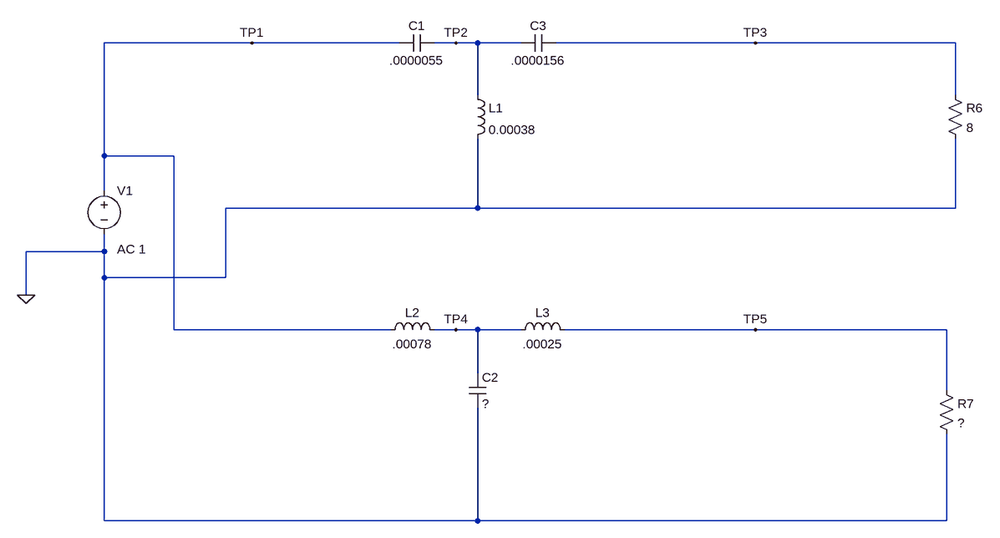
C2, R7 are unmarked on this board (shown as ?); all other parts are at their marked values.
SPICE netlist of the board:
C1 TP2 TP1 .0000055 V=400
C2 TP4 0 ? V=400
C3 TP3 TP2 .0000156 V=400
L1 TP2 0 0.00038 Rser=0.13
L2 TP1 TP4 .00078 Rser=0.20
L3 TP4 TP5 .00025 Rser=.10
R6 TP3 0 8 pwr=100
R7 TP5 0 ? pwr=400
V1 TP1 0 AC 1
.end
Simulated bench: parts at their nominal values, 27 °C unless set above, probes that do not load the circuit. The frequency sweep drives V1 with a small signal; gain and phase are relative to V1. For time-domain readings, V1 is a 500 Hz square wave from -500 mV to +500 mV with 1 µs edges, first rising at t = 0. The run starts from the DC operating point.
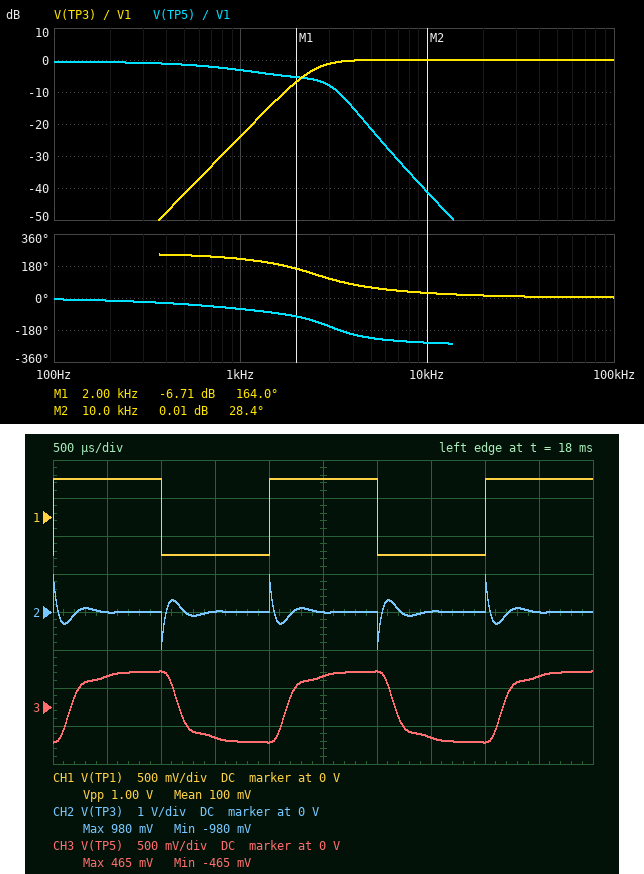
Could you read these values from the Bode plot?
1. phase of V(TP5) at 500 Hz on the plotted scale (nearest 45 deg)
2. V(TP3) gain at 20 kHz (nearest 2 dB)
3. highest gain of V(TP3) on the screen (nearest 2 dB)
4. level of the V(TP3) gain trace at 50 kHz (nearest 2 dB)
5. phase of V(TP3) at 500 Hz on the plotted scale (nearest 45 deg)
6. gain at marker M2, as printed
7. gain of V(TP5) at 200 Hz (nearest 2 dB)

-45 deg
0 dB
0 dB
0 dB
225 deg
0.01 dB
0 dB
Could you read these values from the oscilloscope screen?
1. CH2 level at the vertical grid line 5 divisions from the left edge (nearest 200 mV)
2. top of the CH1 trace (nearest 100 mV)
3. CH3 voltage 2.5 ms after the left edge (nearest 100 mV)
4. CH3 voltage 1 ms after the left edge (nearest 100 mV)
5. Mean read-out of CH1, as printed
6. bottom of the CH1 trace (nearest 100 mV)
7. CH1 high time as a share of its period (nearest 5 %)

0 V
500 mV
400 mV
500 mV
100 mV
-500 mV
50 %
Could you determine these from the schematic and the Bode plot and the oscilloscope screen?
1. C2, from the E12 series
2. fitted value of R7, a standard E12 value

12 µF
4.7 Ω
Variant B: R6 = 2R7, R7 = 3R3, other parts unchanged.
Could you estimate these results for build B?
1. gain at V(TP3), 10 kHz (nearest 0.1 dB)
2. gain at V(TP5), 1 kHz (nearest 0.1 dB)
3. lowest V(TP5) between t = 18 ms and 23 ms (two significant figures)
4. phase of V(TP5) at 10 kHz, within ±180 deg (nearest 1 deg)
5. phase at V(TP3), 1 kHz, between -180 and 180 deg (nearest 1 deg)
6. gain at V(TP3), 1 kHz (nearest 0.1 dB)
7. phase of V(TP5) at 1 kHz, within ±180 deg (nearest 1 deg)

-4.4 dB
-5.7 dB
-440 mV
104 deg
-114 deg
-30.5 dB
-69 deg
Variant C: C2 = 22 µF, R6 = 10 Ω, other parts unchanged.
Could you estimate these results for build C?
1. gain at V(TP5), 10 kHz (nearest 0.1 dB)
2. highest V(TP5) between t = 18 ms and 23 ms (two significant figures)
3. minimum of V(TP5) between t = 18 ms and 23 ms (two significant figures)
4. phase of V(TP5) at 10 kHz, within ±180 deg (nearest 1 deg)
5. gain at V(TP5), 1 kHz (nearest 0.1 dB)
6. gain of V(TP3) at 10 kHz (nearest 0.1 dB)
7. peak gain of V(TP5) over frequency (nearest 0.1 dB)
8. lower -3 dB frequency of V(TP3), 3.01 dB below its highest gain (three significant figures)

-47.0 dB
480 mV
-480 mV
108 deg
-1.8 dB
0.4 dB
-0.5 dB
2.59 kHz
